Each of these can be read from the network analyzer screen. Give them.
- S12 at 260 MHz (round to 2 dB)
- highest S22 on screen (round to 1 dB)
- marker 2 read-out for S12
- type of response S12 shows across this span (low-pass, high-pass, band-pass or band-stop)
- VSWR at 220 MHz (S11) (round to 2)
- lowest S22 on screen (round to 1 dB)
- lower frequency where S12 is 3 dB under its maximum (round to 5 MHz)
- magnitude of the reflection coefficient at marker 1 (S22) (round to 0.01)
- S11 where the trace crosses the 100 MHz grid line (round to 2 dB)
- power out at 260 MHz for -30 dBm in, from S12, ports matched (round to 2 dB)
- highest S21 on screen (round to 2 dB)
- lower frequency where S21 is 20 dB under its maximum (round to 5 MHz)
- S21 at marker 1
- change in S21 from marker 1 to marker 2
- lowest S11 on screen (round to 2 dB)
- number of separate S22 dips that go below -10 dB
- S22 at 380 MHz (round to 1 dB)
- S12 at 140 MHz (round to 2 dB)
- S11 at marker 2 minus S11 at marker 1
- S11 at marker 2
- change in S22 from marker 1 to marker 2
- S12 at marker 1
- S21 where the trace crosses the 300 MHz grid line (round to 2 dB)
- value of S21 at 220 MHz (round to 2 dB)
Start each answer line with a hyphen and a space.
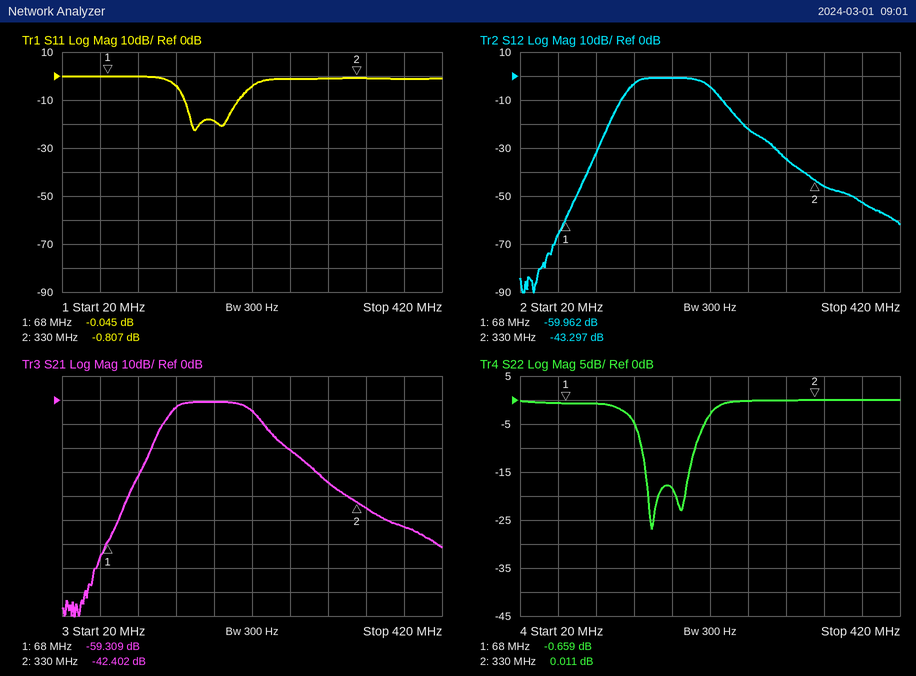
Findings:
- -22 dB
- 0 dB
- -43.297 dB
- band-pass
- 4
- -27 dB
- 140 MHz
- 0.93
- 0 dB
- -52 dBm
- 0 dB
- 115 MHz
- -59.309 dB
- 16.907 dB
- -22 dB
- 2
- 0 dB
- -4 dB
- -0.762 dB
- -0.807 dB
- 0.670 dB
- -59.962 dB
- -34 dB
- -4 dB
